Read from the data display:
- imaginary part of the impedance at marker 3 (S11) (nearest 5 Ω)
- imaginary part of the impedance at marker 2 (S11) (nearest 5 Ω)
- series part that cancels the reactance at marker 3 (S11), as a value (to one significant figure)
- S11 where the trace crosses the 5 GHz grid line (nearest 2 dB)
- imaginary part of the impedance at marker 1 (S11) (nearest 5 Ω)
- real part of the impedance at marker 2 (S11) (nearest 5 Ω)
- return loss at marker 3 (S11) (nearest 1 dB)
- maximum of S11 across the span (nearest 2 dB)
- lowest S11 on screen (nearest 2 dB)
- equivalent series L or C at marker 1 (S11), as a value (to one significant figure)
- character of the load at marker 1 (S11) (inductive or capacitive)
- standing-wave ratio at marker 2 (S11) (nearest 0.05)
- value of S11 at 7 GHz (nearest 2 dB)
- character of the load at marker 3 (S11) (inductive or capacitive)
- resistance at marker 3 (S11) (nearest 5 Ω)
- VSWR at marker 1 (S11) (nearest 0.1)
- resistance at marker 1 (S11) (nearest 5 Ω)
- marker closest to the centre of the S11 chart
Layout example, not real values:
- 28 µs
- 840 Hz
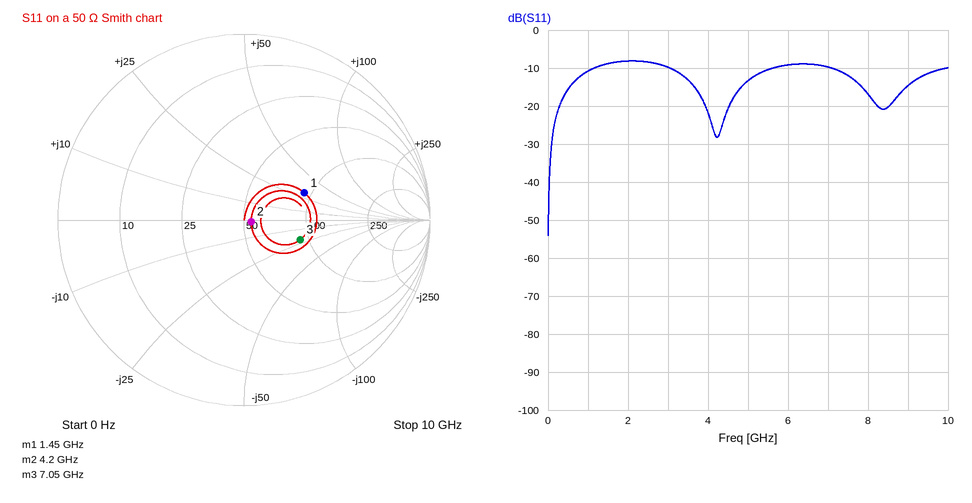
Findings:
- -20 Ω
- 0 Ω
- 500 pH
- -14 dB
- +30 Ω
- 55 Ω
- 10 dB
- -8 dB
- -54 dB
- 3 nH
- inductive
- 1.10
- -10 dB
- capacitive
- 90 Ω
- 2.1
- 90 Ω
- marker 2
